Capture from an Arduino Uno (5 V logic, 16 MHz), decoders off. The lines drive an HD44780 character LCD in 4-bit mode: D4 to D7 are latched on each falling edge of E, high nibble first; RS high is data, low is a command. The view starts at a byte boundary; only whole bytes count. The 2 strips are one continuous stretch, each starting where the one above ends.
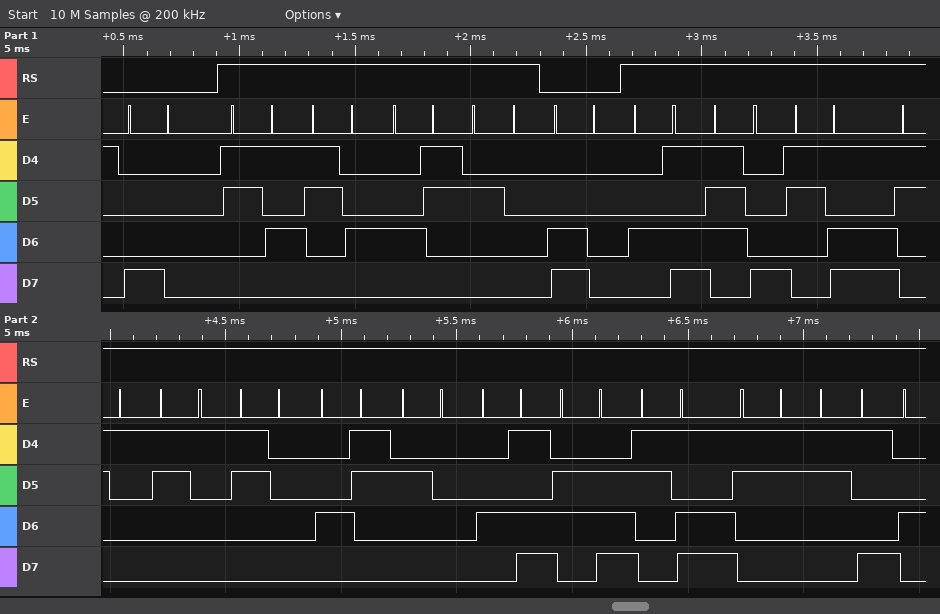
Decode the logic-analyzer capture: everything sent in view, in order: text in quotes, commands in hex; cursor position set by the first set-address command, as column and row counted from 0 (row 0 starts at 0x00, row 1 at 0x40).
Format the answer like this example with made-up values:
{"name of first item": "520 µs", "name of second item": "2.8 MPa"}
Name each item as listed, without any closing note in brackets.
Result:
{"everything sent in view, in order: text in quotes, commands in hex": "0x80 \"54C \" 0xC0 \"Mx=110C Mn=39\"", "cursor position set by the first set-address command, as column and row counted from 0": "column 0, row 0"}
